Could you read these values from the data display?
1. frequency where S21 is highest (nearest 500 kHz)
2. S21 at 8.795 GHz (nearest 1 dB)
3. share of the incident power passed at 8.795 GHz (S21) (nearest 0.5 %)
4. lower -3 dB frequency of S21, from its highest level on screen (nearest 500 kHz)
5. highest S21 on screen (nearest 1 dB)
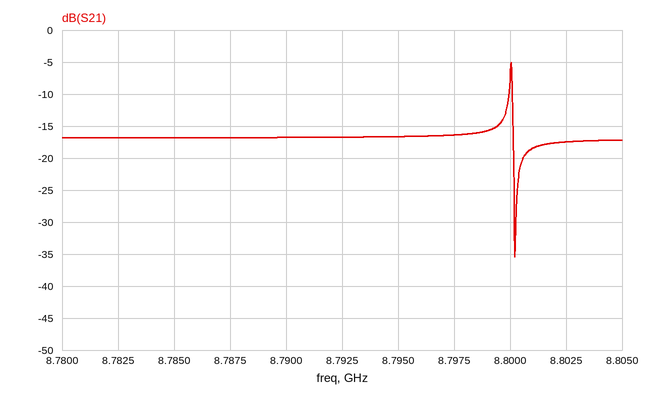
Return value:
8.8000 GHz
-17 dB
2.0 %
8.8000 GHz
-5 dB
